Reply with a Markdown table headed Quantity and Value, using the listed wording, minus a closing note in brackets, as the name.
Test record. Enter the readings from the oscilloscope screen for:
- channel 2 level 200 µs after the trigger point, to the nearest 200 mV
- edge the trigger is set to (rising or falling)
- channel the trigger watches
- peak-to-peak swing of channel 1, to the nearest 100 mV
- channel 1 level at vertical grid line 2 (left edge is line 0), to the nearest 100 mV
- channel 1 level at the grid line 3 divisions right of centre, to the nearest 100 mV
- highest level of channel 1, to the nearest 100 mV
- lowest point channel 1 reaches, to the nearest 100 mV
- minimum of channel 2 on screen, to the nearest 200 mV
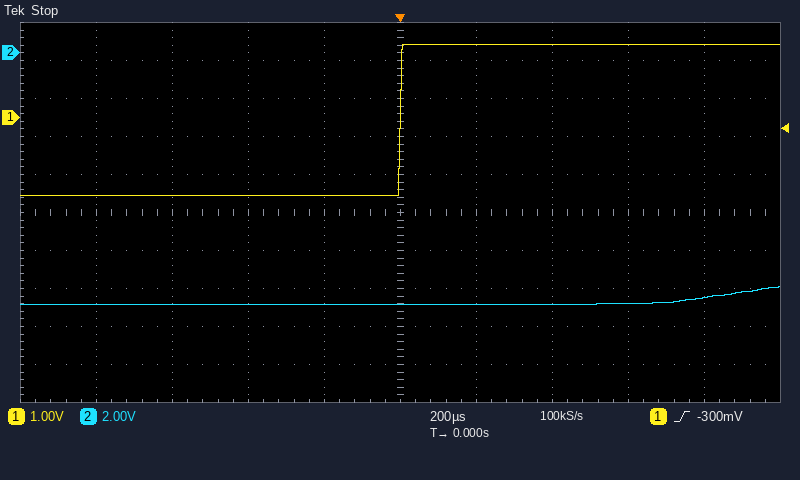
| Quantity | Value |
|---|---|
| channel 2 level 200 µs after the trigger point, to the nearest 200 mV | -13.2 V |
| edge the trigger is set to | rising |
| channel the trigger watches | channel 1 |
| peak-to-peak swing of channel 1, to the nearest 100 mV | 4.0 V |
| channel 1 level at vertical grid line 2 (left edge is line 0), to the nearest 100 mV | -2.1 V |
| channel 1 level at the grid line 3 divisions right of centre, to the nearest 100 mV | 1.9 V |
| highest level of channel 1, to the nearest 100 mV | 1.9 V |
| lowest point channel 1 reaches, to the nearest 100 mV | -2.1 V |
| minimum of channel 2 on screen, to the nearest 200 mV | -13.2 V |
